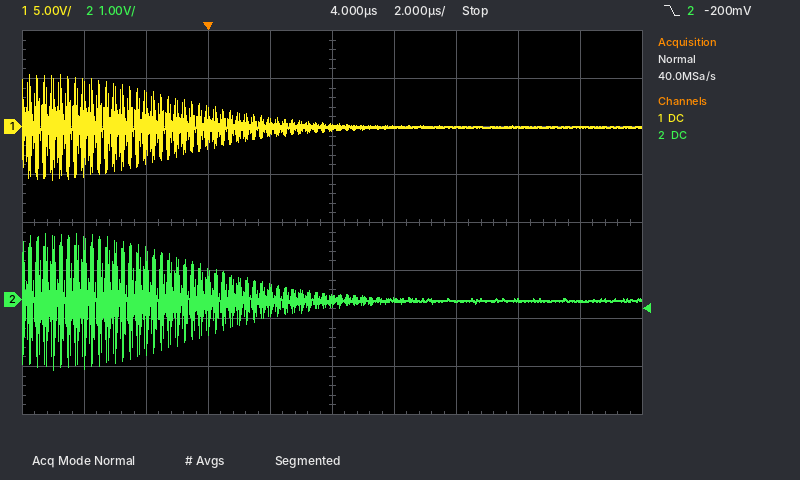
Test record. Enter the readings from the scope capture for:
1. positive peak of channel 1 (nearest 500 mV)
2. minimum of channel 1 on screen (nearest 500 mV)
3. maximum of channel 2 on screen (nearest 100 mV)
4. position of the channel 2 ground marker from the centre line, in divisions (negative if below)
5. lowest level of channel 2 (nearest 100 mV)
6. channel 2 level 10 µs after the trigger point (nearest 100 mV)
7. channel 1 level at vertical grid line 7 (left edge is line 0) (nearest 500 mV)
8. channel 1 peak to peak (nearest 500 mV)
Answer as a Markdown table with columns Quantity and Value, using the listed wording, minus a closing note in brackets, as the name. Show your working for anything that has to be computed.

| Quantity | Value |
|---|---|
| positive peak of channel 1 | 5.5 V |
| minimum of channel 1 on screen | -5.5 V |
| maximum of channel 2 on screen | 1.4 V |
| position of the channel 2 ground marker from the centre line, in divisions | -1.6 div |
| lowest level of channel 2 | -1.5 V |
| channel 2 level 10 µs after the trigger point | 0.0 V |
| channel 1 level at vertical grid line 7 (left edge is line 0) | 0.0 V |
| channel 1 peak to peak | 5.5 V − (-5.5 V) = 11.0 V |
